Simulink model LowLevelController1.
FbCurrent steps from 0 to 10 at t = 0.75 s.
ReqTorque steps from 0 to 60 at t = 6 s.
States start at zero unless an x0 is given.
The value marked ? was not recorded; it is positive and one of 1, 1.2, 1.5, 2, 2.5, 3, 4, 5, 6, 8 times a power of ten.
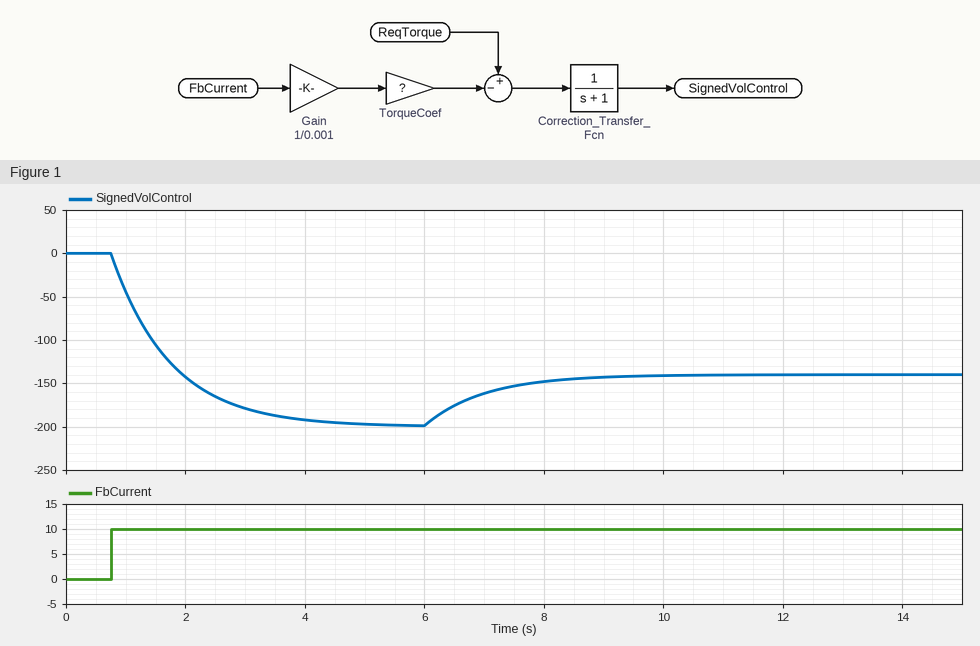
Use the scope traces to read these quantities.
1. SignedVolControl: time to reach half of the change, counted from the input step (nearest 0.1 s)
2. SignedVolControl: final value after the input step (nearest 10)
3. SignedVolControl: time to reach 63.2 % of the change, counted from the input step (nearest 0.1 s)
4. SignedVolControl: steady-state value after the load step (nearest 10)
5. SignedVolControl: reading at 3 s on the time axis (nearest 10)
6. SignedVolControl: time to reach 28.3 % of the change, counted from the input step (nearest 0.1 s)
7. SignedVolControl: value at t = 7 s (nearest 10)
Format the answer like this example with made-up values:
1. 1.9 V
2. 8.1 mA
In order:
1. 0.7 s
2. -200
3. 1.0 s
4. -140
5. -180
6. 0.3 s
7. -160
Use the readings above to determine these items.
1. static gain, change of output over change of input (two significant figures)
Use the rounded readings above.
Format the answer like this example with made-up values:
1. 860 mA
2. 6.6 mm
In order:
1. -20
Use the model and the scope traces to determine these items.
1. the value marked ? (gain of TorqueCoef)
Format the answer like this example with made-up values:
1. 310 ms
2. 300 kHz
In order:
1. 0.02
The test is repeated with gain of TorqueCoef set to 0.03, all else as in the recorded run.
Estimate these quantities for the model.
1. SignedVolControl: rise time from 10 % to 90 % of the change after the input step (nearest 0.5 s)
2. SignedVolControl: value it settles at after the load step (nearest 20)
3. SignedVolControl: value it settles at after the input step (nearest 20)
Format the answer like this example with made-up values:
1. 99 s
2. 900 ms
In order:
1. 2.0 s
2. -240
3. -300
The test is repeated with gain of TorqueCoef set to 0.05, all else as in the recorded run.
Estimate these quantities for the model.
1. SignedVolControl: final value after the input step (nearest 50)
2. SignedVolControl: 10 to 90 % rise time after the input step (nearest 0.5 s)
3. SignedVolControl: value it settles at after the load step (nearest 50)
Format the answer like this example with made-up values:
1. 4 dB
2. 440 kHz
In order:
1. -500
2. 2.0 s
3. -450
